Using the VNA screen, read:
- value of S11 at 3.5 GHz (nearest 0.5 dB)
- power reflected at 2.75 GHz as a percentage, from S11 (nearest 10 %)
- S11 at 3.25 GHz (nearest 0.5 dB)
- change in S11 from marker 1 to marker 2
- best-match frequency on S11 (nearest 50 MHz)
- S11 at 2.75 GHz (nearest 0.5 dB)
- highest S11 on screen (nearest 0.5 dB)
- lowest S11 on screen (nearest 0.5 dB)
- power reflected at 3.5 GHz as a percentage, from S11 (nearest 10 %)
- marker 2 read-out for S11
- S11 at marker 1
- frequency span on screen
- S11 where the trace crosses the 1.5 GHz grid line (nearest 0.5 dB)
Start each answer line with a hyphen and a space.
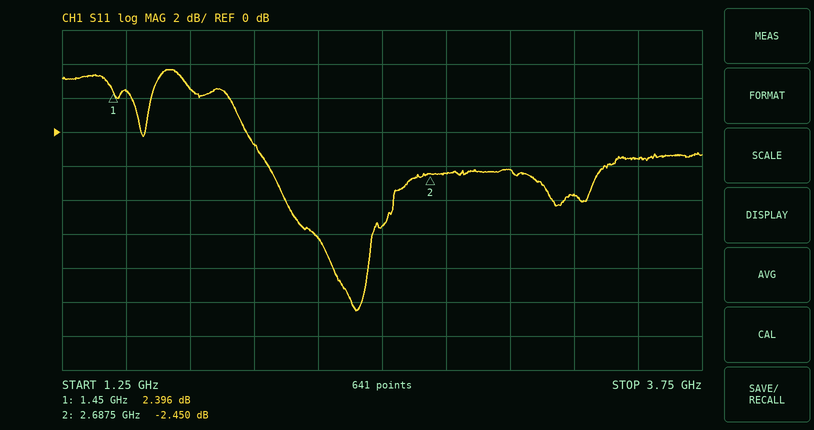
- -1.5 dB
- 60 %
- -3.5 dB
- -4.846 dB
- 2.40 GHz
- -2.5 dB
- 3.5 dB
- -10.5 dB
- 70 %
- -2.450 dB
- 2.396 dB
- 2.5 GHz
- 2.5 dB
